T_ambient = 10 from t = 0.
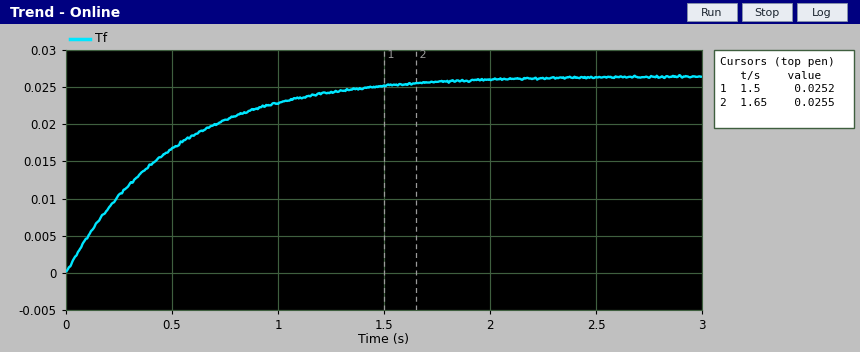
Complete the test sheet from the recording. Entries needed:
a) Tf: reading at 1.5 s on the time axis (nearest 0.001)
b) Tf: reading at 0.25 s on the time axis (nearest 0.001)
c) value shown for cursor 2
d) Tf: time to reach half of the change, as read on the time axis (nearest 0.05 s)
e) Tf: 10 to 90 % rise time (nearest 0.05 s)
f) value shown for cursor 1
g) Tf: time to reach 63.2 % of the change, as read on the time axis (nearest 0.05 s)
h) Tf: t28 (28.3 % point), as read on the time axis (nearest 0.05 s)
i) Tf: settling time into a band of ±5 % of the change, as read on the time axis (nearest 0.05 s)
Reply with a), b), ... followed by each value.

a) 0.025
b) 0.010
c) 0.0255
d) 0.35 s
e) 1.10 s
f) 0.0252
g) 0.50 s
h) 0.15 s
i) 1.50 s
